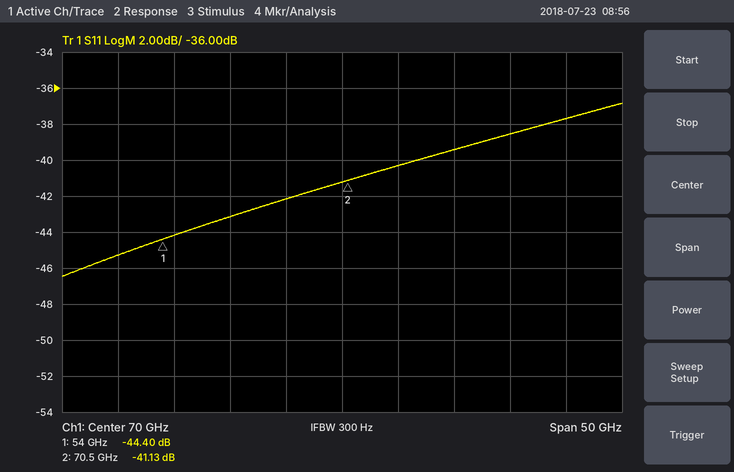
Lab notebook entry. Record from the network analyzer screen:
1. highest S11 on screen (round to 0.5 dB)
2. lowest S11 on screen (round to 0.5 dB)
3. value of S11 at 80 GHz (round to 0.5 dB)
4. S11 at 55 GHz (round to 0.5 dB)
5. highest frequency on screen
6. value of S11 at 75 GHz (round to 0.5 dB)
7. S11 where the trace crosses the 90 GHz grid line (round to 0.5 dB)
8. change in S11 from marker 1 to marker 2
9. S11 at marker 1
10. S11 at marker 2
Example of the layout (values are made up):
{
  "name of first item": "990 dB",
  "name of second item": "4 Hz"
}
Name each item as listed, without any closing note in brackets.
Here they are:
{
  "highest S11 on screen": "-37.0 dB",
  "lowest S11 on screen": "-46.5 dB",
  "value of S11 at 80 GHz": "-39.5 dB",
  "S11 at 55 GHz": "-44.0 dB",
  "highest frequency on screen": "95 GHz",
  "value of S11 at 75 GHz": "-40.5 dB",
  "S11 where the trace crosses the 90 GHz grid line": "-37.5 dB",
  "change in S11 from marker 1 to marker 2": "3.27 dB",
  "S11 at marker 1": "-44.40 dB",
  "S11 at marker 2": "-41.13 dB"
}
